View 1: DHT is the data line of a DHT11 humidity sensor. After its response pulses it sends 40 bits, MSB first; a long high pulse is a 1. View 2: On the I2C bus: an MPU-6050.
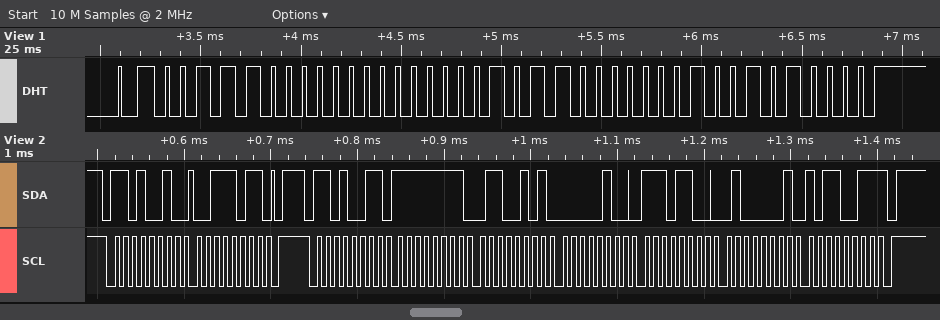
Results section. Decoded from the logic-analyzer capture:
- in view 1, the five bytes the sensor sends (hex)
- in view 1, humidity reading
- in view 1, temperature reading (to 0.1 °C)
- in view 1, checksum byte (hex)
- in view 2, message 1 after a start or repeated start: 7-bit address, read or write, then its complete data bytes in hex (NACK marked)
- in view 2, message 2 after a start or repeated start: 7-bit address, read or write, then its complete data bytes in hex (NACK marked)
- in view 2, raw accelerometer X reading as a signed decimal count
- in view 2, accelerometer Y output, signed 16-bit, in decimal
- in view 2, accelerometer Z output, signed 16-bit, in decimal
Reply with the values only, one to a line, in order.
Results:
38 00 16 02 50
56 %
22.2 °C
0x50
0x69 write: 3B
0x69 read: FF 65 04 EC 41 B3 NACK
-155
1260
16819
